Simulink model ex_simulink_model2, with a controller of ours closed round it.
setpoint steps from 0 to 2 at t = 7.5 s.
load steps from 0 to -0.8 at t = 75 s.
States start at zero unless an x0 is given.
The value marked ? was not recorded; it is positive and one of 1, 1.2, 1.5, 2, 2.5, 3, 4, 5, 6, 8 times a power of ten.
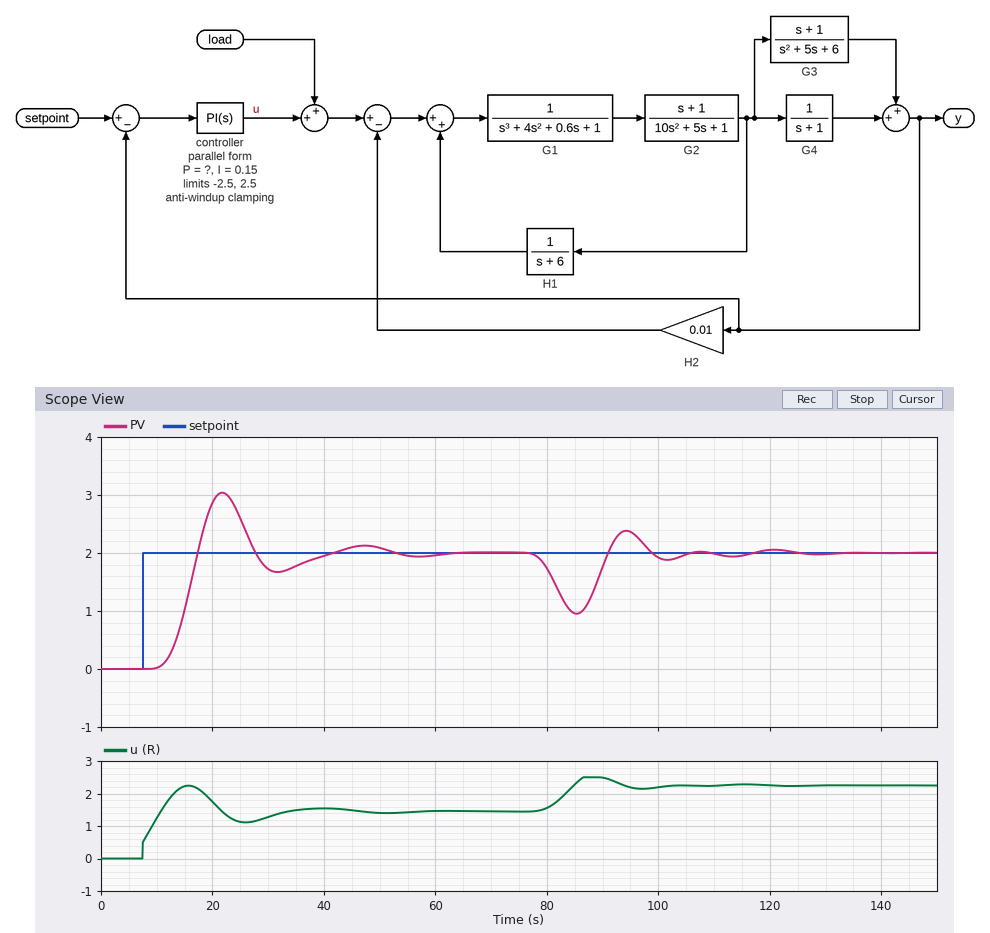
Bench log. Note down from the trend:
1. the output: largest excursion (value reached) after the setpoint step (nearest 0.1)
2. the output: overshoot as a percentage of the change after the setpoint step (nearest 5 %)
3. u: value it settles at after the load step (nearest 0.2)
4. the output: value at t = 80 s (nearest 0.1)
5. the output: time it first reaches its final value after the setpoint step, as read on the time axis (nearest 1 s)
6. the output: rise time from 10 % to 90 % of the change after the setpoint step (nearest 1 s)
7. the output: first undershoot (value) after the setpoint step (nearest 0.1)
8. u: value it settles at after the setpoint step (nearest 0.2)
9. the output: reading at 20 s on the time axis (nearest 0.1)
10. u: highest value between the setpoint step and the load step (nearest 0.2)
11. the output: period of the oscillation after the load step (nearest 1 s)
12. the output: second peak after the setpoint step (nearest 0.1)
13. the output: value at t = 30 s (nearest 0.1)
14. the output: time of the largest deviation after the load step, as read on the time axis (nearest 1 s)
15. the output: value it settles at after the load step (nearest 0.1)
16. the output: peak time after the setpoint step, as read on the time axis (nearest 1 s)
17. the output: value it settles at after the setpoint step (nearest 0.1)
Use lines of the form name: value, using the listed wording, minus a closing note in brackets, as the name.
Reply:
the output: largest excursion (value reached) after the setpoint step: 3.0
the output: overshoot as a percentage of the change after the setpoint step: 50 %
u: value it settles at after the load step: 2.2
the output: value at t = 80 s: 1.7
the output: time it first reaches its final value after the setpoint step, as read on the time axis: 17 s
the output: rise time from 10 % to 90 % of the change after the setpoint step: 5 s
the output: first undershoot (value) after the setpoint step: 1.7
u: value it settles at after the setpoint step: 1.4
the output: reading at 20 s on the time axis: 2.9
u: highest value between the setpoint step and the load step: 2.2
the output: period of the oscillation after the load step: 16 s
the output: second peak after the setpoint step: 2.1
the output: value at t = 30 s: 1.7
the output: time of the largest deviation after the load step, as read on the time axis: 85 s
the output: value it settles at after the load step: 2.0
the output: peak time after the setpoint step, as read on the time axis: 22 s
the output: value it settles at after the setpoint step: 2.0
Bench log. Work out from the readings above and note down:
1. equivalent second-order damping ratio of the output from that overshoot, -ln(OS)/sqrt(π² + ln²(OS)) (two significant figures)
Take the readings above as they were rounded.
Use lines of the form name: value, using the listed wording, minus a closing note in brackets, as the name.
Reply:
equivalent second-order damping ratio of the output from that overshoot, -ln(OS)/sqrt(π² + ln²(OS)): 0.22
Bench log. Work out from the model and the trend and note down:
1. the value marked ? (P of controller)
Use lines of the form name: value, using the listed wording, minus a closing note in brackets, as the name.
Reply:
the value marked ?: 0.25
